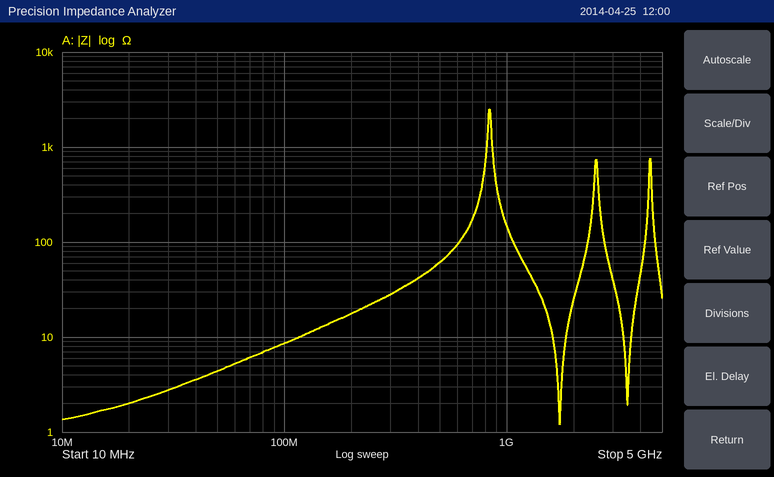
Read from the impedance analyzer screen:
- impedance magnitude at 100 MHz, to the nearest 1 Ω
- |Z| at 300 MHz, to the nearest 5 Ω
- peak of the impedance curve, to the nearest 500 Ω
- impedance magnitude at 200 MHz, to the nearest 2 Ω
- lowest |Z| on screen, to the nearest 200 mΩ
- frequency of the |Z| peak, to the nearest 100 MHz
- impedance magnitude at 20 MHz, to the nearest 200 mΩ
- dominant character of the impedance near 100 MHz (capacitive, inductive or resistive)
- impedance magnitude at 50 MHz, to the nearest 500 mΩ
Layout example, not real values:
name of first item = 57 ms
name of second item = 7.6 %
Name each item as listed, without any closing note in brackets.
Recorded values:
impedance magnitude at 100 MHz, to the nearest 1 Ω = 9 Ω
|Z| at 300 MHz, to the nearest 5 Ω = 30 Ω
peak of the impedance curve, to the nearest 500 Ω = 2.5 kΩ
impedance magnitude at 200 MHz, to the nearest 2 Ω = 18 Ω
lowest |Z| on screen, to the nearest 200 mΩ = 1.2 Ω
frequency of the |Z| peak, to the nearest 100 MHz = 800 MHz
impedance magnitude at 20 MHz, to the nearest 200 mΩ = 2.0 Ω
dominant character of the impedance near 100 MHz = inductive
impedance magnitude at 50 MHz, to the nearest 500 mΩ = 4.5 Ω
